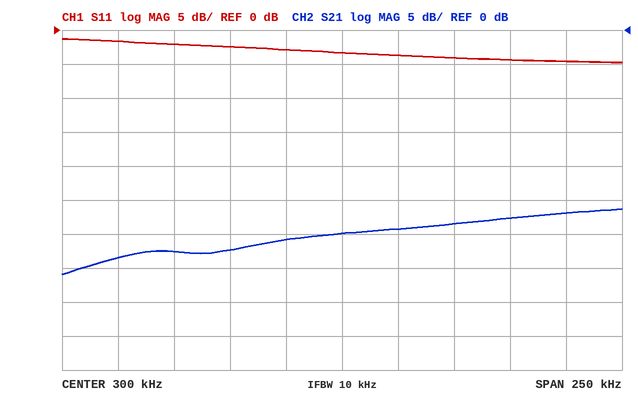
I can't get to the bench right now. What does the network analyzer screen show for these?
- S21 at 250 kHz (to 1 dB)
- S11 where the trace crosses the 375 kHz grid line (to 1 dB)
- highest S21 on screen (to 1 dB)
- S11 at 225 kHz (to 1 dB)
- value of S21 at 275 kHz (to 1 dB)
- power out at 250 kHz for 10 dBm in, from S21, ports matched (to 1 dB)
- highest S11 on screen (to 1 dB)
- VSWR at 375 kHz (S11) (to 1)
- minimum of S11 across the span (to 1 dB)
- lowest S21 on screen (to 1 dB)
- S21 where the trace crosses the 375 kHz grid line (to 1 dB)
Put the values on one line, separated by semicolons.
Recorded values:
-32 dB; -4 dB; -26 dB; -2 dB; -31 dB; -22 dBm; -1 dB; 4; -5 dB; -36 dB; -28 dB
